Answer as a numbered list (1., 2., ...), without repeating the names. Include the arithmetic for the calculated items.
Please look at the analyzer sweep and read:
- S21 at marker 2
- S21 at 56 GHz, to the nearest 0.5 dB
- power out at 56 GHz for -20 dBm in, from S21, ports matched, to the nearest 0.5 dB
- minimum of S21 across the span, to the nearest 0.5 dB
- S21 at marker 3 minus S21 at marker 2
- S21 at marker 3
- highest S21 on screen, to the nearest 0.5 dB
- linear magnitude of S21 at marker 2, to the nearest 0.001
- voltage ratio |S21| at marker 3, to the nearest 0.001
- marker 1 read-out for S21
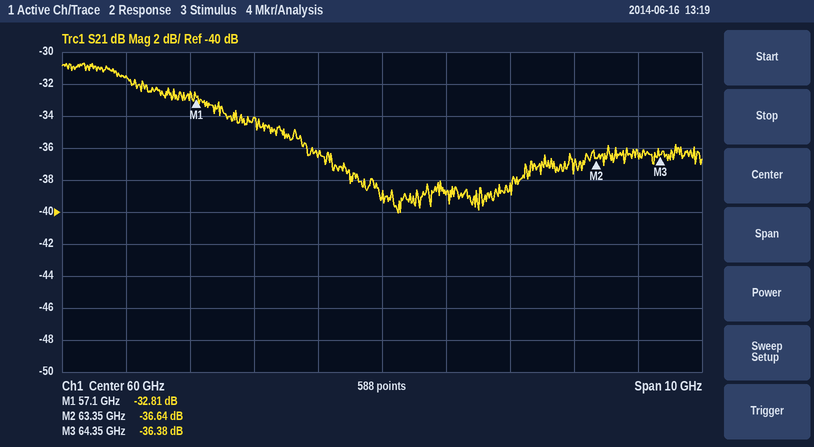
1. -36.64 dB
2. -31.5 dB
3. -20 dBm + (-31.5 dB) = -51.5 dBm
4. -40.0 dB
5. -36.38 − (-36.64) = 0.26 dB
6. -36.38 dB
7. -30.5 dB
8. 10^(-36.64/20) ≈ 0.015
9. 10^(-36.38/20) ≈ 0.015
10. -32.81 dB
